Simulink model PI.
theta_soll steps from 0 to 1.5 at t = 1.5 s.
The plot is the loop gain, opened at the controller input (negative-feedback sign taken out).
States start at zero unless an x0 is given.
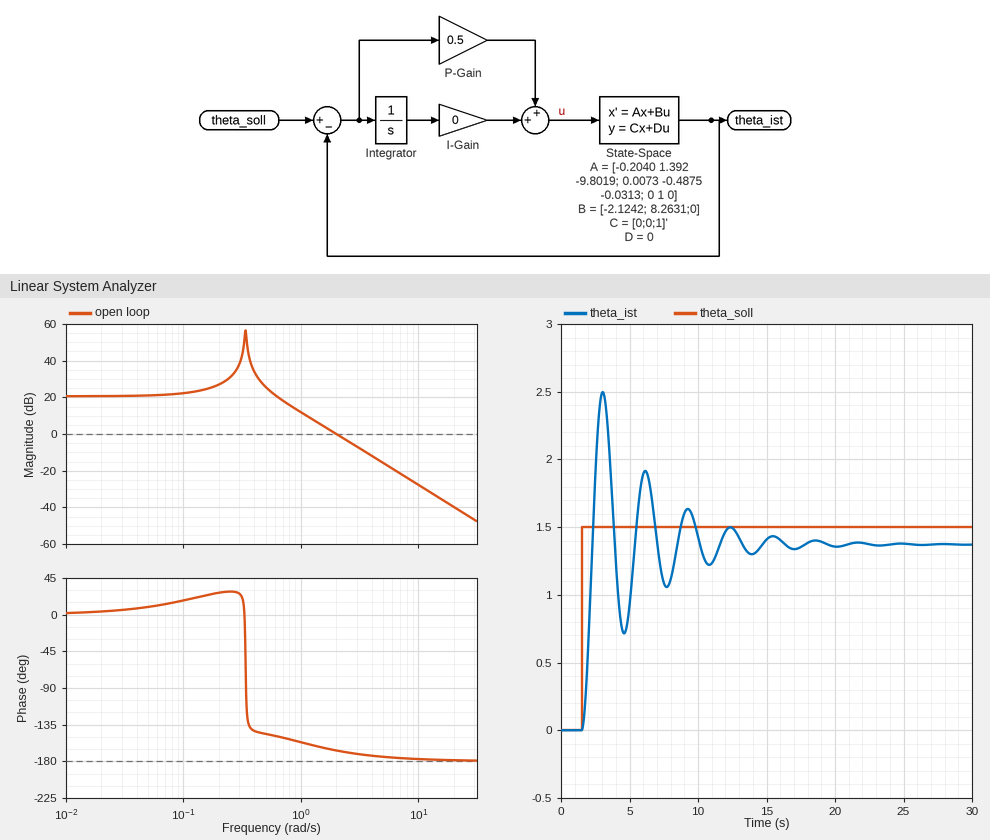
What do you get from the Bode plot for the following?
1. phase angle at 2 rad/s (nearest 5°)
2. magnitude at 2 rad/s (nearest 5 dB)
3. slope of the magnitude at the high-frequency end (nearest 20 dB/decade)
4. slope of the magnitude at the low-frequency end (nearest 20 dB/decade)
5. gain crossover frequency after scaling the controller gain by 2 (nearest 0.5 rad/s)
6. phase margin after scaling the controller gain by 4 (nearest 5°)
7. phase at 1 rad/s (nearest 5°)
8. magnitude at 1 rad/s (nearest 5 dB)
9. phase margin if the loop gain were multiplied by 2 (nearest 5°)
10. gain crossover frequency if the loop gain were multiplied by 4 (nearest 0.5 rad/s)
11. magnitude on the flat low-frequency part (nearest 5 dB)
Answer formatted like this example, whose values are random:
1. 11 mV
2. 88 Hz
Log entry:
1. -165°
2. 0 dB
3. -40 dB/decade
4. 0 dB/decade
5. 3.0 rad/s
6. 5°
7. -155°
8. 10 dB
9. 10°
10. 4.0 rad/s
11. 20 dB
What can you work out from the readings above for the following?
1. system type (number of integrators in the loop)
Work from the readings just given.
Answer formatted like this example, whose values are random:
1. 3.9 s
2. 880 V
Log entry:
1. 0
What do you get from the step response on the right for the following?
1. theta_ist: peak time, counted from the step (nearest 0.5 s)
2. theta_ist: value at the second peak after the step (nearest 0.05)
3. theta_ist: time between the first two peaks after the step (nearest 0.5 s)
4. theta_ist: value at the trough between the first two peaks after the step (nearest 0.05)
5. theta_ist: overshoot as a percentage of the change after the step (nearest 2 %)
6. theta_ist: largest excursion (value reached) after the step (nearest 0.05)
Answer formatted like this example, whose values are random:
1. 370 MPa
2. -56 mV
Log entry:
1. 1.5 s
2. 1.90
3. 3.0 s
4. 0.70
5. 82 %
6. 2.50
